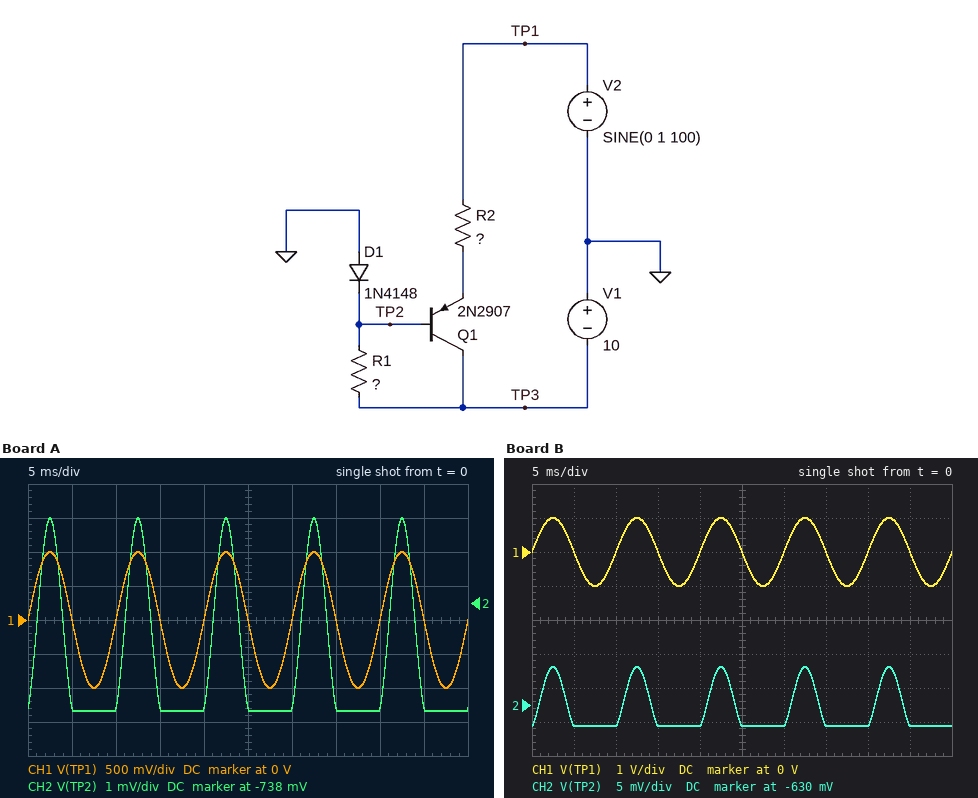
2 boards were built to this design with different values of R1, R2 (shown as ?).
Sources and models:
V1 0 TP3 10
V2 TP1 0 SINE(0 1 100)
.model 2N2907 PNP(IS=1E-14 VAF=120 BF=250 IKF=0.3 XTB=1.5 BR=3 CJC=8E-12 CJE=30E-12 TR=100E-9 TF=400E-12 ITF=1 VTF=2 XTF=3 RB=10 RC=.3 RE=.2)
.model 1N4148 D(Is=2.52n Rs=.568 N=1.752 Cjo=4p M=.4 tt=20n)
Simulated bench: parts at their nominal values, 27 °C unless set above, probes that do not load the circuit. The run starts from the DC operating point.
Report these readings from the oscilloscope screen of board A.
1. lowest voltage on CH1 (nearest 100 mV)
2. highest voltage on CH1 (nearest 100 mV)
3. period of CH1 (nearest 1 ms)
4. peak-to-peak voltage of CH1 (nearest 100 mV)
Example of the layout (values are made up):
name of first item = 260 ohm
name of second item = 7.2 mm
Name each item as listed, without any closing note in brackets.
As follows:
lowest voltage on CH1 = -1.0 V
highest voltage on CH1 = 1.0 V
period of CH1 = 10 ms
peak-to-peak voltage of CH1 = 2.0 V
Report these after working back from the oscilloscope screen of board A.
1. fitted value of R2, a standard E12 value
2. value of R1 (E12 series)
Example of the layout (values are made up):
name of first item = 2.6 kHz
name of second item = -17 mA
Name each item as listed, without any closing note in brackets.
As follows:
fitted value of R2, a standard E12 value = 2.7 Ω
value of R1 = 390 Ω
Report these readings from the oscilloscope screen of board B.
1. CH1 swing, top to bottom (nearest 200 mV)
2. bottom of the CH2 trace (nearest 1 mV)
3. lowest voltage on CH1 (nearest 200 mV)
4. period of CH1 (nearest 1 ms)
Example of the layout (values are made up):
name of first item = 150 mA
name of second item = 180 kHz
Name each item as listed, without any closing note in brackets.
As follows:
CH1 swing, top to bottom = 2.0 V
bottom of the CH2 trace = -633 mV
lowest voltage on CH1 = -1.0 V
period of CH1 = 10 ms
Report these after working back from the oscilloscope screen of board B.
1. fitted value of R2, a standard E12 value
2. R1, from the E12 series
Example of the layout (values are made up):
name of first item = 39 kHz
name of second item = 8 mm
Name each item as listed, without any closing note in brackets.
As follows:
fitted value of R2, a standard E12 value = 8.2 Ω
R1, from the E12 series = 3.3 kΩ
